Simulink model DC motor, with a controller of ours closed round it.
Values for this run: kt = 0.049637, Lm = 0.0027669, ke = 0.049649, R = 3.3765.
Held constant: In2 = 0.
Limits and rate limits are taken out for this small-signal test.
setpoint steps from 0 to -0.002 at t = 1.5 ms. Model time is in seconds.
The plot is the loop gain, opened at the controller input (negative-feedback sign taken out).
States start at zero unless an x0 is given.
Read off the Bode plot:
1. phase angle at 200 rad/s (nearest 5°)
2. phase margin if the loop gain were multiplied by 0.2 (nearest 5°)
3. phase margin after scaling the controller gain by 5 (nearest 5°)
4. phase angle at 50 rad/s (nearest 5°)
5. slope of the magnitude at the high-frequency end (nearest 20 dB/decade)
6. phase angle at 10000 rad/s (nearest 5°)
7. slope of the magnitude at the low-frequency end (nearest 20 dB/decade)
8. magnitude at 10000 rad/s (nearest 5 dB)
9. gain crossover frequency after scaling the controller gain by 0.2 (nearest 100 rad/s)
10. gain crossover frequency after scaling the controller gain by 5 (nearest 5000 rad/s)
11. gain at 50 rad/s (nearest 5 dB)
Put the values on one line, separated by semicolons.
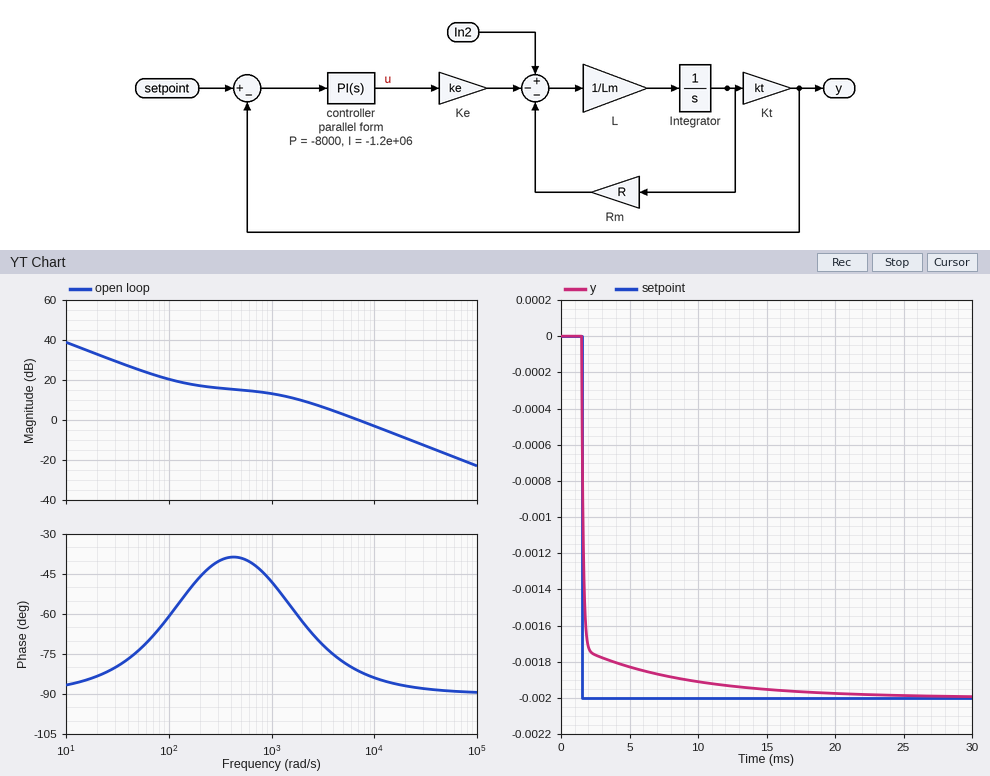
-45°; 135°; 90°; -75°; -20 dB/decade; -85°; -20 dB/decade; -5 dB; 800 rad/s; 35000 rad/s; 25 dB
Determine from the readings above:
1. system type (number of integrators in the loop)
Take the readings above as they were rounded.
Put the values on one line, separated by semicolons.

1
